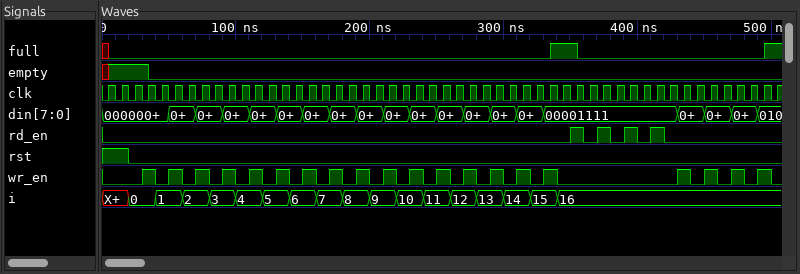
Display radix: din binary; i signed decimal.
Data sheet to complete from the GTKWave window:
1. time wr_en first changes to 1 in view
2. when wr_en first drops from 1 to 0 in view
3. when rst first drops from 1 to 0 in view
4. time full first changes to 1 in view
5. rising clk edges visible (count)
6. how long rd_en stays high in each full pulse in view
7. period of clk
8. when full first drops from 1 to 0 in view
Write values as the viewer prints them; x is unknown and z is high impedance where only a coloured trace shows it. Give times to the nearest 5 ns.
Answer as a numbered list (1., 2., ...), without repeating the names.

1. 30 ns
2. 40 ns
3. 20 ns
4. 335 ns
5. 51
6. 10 ns, 10 ns, 10 ns, 10 ns
7. 10 ns
8. 355 ns
